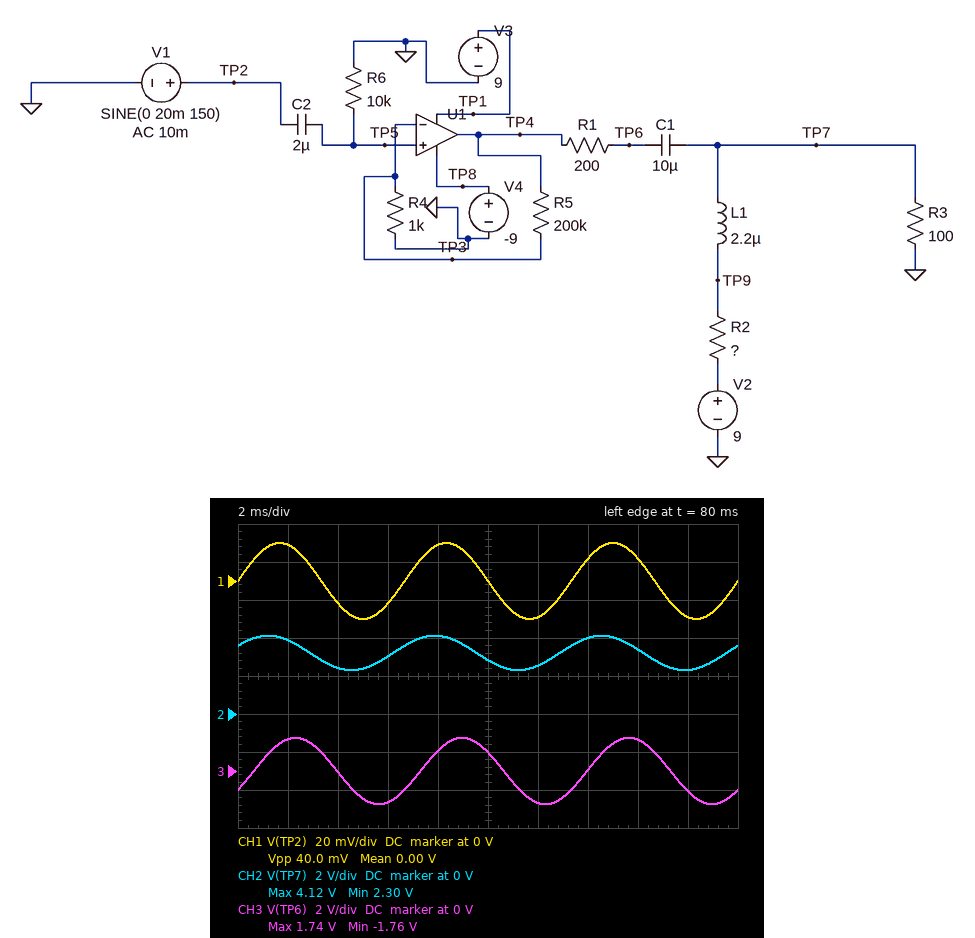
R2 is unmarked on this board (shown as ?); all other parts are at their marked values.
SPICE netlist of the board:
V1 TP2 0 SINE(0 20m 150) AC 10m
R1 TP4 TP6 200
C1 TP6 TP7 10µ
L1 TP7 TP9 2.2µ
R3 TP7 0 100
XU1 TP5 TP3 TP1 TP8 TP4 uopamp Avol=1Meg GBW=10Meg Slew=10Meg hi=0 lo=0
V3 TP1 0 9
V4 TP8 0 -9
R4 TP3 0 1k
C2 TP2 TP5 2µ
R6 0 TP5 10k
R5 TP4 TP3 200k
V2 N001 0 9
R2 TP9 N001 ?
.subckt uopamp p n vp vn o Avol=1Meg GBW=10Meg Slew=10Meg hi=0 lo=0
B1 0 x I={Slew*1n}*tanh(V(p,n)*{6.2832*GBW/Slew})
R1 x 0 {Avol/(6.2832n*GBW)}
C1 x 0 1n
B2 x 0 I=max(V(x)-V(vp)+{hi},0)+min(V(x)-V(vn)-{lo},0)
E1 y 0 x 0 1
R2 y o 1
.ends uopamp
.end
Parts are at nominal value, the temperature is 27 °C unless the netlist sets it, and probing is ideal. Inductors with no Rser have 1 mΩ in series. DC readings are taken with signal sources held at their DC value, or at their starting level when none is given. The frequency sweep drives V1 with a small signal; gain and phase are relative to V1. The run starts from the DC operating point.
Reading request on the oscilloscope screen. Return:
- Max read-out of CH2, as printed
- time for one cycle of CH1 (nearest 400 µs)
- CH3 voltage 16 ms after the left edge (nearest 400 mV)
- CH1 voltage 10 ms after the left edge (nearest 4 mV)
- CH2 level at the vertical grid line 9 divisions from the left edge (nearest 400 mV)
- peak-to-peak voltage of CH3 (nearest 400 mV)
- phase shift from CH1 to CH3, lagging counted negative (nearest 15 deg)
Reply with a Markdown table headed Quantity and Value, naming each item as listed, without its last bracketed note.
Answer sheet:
| Quantity | Value |
|---|---|
| Max read-out of CH2, as printed | 4.12 V |
| time for one cycle of CH1 | 6.8 ms |
| CH3 voltage 16 ms after the left edge | 1.6 V |
| CH1 voltage 10 ms after the left edge | 0 V |
| CH2 level at the vertical grid line 9 divisions from the left edge | 2.4 V |
| peak-to-peak voltage of CH3 | 3.6 V |
| phase shift from CH1 to CH3, lagging counted negative | -30 deg |
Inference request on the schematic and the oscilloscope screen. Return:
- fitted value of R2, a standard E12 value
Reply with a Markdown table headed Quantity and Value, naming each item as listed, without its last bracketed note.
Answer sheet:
| Quantity | Value |
|---|---|
| fitted value of R2, a standard E12 value | 180 Ω |
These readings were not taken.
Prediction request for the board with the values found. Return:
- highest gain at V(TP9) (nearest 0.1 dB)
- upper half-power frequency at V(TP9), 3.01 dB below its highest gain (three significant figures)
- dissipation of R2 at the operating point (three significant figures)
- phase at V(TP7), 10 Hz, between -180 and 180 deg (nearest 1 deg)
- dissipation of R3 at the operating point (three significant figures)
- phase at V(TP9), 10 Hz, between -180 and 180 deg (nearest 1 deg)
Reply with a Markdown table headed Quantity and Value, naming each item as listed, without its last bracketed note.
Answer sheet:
| Quantity | Value |
|---|---|
| highest gain at V(TP9) | 33.8 dB |
| upper half-power frequency at V(TP9), 3.01 dB below its highest gain | 49.7 kHz |
| dissipation of R2 at the operating point | 186 mW |
| phase at V(TP7), 10 Hz, between -180 and 180 deg | 119 deg |
| dissipation of R3 at the operating point | 103 mW |
| phase at V(TP9), 10 Hz, between -180 and 180 deg | 119 deg |
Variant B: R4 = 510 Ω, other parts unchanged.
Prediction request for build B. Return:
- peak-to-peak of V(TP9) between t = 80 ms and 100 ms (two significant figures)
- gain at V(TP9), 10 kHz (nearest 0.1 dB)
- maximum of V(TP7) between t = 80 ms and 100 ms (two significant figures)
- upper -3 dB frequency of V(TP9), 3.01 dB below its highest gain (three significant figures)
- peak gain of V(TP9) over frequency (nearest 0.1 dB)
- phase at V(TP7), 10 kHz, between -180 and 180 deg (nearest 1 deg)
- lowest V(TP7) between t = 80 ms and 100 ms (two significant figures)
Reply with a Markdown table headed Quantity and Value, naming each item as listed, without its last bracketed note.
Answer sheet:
| Quantity | Value |
|---|---|
| peak-to-peak of V(TP9) between t = 80 ms and 100 ms | 3.5 V |
| gain at V(TP9), 10 kHz | 39.0 dB |
| maximum of V(TP7) between t = 80 ms and 100 ms | 5.0 V |
| upper -3 dB frequency of V(TP9), 3.01 dB below its highest gain | 25.5 kHz |
| peak gain of V(TP9) over frequency | 39.6 dB |
| phase at V(TP7), 10 kHz, between -180 and 180 deg | -21 deg |
| lowest V(TP7) between t = 80 ms and 100 ms | 1.4 V |
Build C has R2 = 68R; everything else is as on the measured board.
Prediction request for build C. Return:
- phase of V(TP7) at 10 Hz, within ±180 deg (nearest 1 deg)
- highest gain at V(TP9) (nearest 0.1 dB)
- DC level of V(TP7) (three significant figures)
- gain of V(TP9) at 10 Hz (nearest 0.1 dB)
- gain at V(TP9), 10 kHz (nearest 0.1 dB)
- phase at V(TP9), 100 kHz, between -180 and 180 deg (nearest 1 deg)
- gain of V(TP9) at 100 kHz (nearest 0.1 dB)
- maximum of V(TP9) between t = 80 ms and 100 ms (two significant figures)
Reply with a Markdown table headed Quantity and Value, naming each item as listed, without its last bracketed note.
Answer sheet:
| Quantity | Value |
|---|---|
| phase of V(TP7) at 10 Hz, within ±180 deg | 120 deg |
| highest gain at V(TP9) | 30.6 dB |
| DC level of V(TP7) | 5.36 V |
| gain of V(TP9) at 10 Hz | 11.9 dB |
| gain at V(TP9), 10 kHz | 30.4 dB |
| phase at V(TP9), 100 kHz, between -180 and 180 deg | -64 deg |
| gain of V(TP9) at 100 kHz | 23.5 dB |
| maximum of V(TP9) between t = 80 ms and 100 ms | 6.0 V |
